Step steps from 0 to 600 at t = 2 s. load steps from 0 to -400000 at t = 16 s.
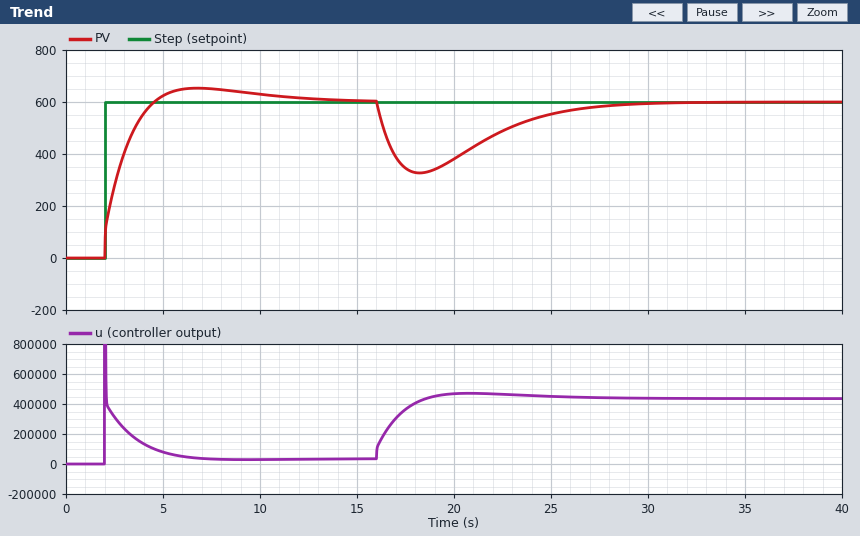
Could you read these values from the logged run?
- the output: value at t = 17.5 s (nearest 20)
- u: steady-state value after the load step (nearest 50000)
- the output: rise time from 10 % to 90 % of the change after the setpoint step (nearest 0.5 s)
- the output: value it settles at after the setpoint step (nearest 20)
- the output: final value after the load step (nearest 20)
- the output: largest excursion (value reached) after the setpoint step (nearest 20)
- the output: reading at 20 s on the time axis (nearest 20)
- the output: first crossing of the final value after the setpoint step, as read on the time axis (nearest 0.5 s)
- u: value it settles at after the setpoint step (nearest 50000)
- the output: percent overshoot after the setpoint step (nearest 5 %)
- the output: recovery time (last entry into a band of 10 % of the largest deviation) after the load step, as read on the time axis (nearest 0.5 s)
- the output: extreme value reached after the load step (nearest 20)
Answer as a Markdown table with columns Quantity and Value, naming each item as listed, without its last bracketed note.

| Quantity | Value |
|---|---|
| the output: value at t = 17.5 s | 340 |
| u: steady-state value after the load step | 450000 |
| the output: rise time from 10 % to 90 % of the change after the setpoint step | 2.0 s |
| the output: value it settles at after the setpoint step | 600 |
| the output: final value after the load step | 600 |
| the output: largest excursion (value reached) after the setpoint step | 660 |
| the output: reading at 20 s on the time axis | 380 |
| the output: first crossing of the final value after the setpoint step, as read on the time axis | 4.5 s |
| u: value it settles at after the setpoint step | 50000 |
| the output: percent overshoot after the setpoint step | 10 % |
| the output: recovery time (last entry into a band of 10 % of the largest deviation) after the load step, as read on the time axis | 26.5 s |
| the output: extreme value reached after the load step | 320 |
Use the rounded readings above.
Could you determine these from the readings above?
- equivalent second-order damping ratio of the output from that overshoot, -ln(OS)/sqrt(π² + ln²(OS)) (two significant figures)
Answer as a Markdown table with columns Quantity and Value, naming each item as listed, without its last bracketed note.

| Quantity | Value |
|---|---|
| equivalent second-order damping ratio of the output from that overshoot, -ln(OS)/sqrt(π² + ln²(OS)) | 0.59 |
